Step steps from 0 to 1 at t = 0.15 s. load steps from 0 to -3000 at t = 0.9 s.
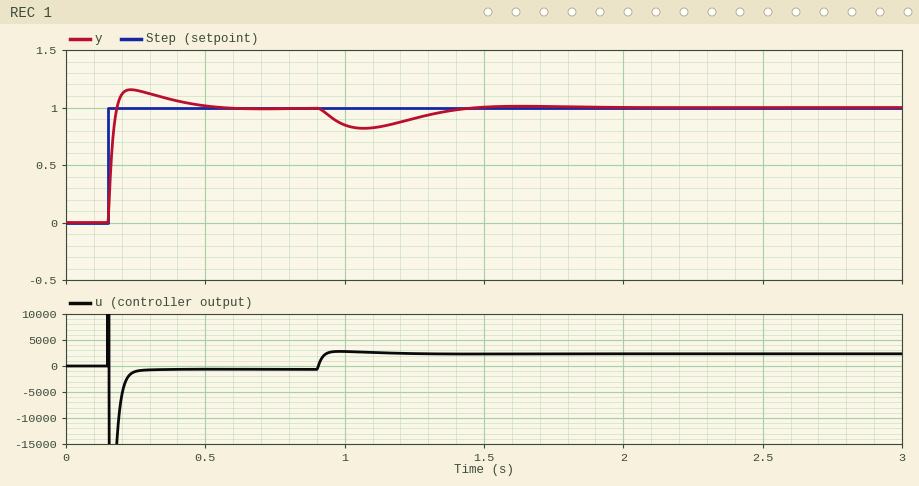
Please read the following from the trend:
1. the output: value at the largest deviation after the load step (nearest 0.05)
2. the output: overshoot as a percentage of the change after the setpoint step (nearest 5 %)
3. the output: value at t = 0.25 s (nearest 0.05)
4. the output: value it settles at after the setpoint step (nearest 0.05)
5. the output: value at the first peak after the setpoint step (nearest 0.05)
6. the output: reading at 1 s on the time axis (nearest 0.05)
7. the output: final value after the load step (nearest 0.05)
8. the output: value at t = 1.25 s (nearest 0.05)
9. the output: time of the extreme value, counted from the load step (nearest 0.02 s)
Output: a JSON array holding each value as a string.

["0.80", "15 %", "1.15", "1.00", "1.15", "0.85", "1.00", "0.90", "0.16 s"]
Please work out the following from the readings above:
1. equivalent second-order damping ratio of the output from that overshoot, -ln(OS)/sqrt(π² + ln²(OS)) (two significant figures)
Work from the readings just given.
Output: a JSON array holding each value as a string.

["0.52"]
